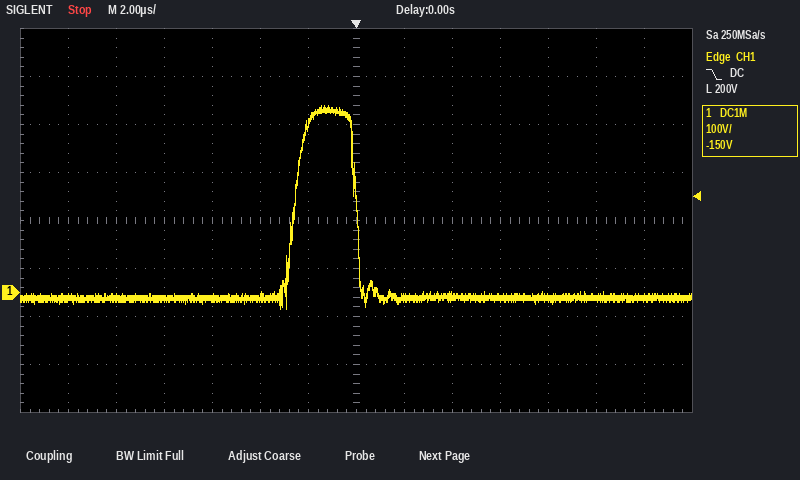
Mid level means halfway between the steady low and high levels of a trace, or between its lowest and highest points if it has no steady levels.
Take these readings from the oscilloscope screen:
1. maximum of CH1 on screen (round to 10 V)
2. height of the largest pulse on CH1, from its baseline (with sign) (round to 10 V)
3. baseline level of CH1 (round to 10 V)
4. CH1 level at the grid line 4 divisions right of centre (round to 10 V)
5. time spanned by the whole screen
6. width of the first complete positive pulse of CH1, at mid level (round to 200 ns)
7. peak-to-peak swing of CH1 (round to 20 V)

390 V
+400 V
-10 V
-10 V
28 µs
2.6 µs
420 V
